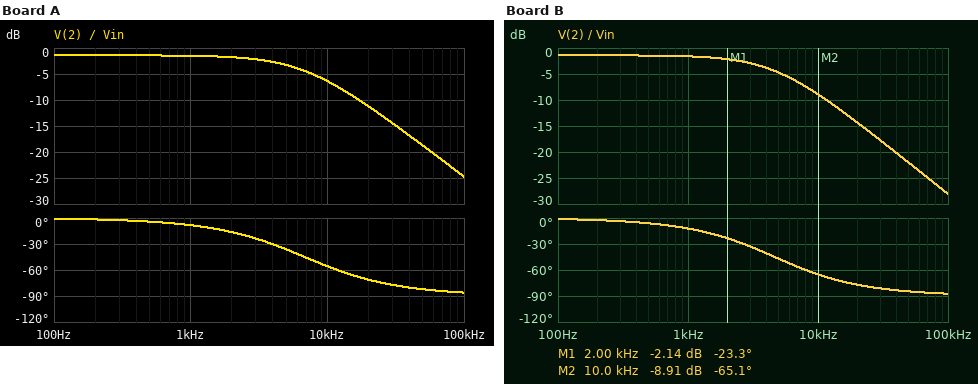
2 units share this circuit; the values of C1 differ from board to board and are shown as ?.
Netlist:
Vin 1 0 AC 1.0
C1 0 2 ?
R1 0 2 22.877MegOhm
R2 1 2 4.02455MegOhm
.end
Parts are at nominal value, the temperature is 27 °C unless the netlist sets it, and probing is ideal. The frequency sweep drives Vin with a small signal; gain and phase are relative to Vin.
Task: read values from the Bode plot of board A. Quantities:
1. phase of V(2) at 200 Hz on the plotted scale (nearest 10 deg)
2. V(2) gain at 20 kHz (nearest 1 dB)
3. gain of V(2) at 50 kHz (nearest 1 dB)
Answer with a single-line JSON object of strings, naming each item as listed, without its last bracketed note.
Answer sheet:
{"phase of V(2) at 200 Hz on the plotted scale": "0 deg", "V(2) gain at 20 kHz": "-11 dB", "gain of V(2) at 50 kHz": "-19 dB"}
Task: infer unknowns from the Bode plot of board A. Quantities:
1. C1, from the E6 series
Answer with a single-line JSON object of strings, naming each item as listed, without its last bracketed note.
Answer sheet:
{"C1, from the E6 series": "6.8 pF"}
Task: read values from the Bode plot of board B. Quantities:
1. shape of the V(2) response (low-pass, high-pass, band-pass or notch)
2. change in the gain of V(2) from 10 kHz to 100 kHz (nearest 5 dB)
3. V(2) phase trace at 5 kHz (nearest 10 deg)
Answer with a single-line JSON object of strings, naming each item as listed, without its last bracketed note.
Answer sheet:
{"shape of the V(2) response": "low-pass", "change in the gain of V(2) from 10 kHz to 100 kHz": "-20 dB", "V(2) phase trace at 5 kHz": "-50 deg"}
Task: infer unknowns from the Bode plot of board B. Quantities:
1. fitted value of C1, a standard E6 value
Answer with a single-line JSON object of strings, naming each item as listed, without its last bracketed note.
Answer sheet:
{"fitted value of C1, a standard E6 value": "10 pF"}
